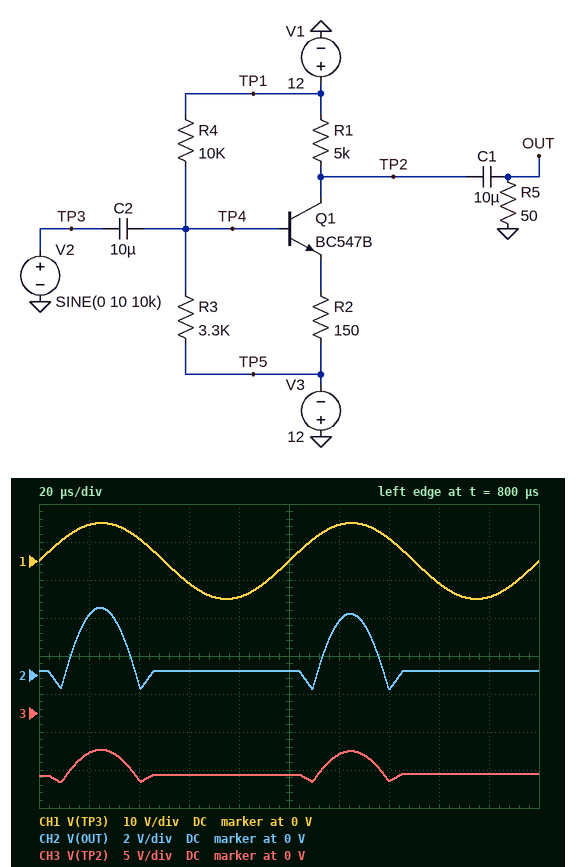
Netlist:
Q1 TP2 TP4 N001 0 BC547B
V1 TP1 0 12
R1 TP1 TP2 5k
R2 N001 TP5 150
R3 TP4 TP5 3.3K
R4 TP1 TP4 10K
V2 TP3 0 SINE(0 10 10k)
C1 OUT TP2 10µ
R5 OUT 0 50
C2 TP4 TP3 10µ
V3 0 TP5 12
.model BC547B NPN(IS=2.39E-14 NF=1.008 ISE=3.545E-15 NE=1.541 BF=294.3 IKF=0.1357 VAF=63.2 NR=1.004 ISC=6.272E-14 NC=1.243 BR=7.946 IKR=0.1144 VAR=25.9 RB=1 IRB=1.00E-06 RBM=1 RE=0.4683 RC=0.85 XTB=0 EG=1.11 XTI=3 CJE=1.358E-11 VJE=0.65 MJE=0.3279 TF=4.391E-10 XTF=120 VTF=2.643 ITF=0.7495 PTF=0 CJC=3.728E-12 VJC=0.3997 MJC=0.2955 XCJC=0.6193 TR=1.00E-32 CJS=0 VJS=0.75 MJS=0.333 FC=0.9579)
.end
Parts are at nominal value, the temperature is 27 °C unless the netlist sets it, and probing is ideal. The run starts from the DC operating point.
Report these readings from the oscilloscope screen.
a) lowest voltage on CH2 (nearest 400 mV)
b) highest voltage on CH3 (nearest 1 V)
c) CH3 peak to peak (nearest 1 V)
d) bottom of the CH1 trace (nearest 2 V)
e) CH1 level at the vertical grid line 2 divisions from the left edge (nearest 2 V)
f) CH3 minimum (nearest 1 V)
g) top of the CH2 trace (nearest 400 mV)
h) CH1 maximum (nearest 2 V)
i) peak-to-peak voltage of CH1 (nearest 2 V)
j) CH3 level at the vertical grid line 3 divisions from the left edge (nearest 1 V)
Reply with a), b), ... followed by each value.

a) -800 mV
b) -5 V
c) 4 V
d) -10 V
e) 6 V
f) -9 V
g) 3.6 V
h) 10 V
i) 20 V
j) -8 V
